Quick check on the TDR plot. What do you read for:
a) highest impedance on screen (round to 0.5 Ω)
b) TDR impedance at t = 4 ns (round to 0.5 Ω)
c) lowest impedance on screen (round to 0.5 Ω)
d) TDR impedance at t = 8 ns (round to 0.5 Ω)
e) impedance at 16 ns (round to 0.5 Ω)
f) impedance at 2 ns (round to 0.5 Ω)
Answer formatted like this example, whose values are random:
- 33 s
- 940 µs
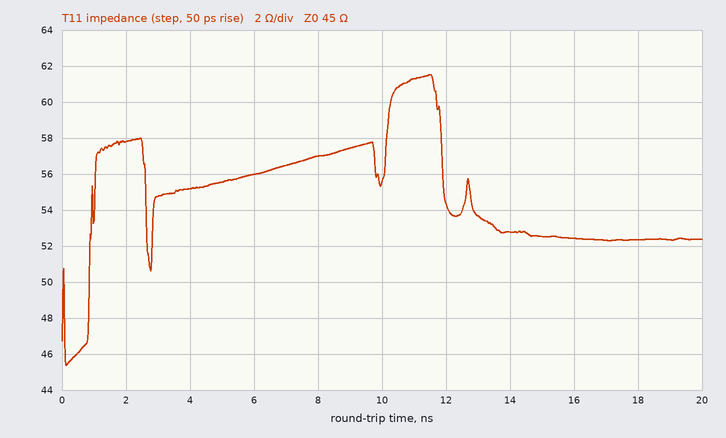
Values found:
- 61.5 Ω
- 55.0 Ω
- 45.5 Ω
- 57.0 Ω
- 52.5 Ω
- 58.0 Ω
